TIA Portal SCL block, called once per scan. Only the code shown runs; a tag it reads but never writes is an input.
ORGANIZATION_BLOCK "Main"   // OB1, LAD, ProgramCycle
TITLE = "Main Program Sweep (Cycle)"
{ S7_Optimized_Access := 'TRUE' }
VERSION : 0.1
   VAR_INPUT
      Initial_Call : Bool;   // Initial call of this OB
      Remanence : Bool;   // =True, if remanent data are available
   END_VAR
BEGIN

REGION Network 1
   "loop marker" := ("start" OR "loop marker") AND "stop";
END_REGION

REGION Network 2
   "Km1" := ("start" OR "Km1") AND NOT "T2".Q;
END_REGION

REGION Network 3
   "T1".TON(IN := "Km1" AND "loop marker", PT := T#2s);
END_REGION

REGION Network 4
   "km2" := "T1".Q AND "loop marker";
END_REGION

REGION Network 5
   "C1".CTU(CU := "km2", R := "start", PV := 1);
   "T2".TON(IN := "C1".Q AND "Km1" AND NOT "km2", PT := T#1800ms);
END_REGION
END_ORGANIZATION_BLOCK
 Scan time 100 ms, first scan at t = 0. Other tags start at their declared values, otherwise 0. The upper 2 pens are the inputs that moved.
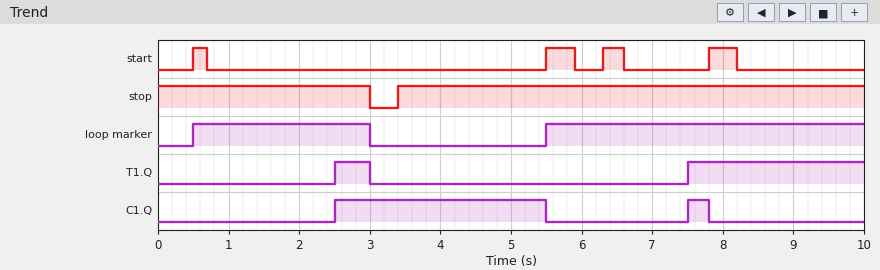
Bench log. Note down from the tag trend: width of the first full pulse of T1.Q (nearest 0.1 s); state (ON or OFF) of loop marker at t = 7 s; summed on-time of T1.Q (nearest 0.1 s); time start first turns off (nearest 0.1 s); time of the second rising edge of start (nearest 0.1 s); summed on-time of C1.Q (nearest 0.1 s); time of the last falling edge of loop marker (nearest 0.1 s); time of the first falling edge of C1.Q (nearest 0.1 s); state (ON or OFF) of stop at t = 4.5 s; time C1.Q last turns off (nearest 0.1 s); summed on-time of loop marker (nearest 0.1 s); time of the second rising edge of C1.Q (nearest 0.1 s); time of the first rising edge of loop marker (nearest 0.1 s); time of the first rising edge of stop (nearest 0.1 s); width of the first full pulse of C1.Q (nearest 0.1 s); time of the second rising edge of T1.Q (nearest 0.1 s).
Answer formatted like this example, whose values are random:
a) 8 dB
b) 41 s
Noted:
a) 0.5 s
b) ON
c) 3.0 s
d) 0.7 s
e) 5.5 s
f) 3.3 s
g) 3.0 s
h) 5.5 s
i) ON
j) 7.8 s
k) 7.0 s
l) 7.5 s
m) 0.5 s
n) 3.4 s
o) 3.0 s
p) 7.5 s
